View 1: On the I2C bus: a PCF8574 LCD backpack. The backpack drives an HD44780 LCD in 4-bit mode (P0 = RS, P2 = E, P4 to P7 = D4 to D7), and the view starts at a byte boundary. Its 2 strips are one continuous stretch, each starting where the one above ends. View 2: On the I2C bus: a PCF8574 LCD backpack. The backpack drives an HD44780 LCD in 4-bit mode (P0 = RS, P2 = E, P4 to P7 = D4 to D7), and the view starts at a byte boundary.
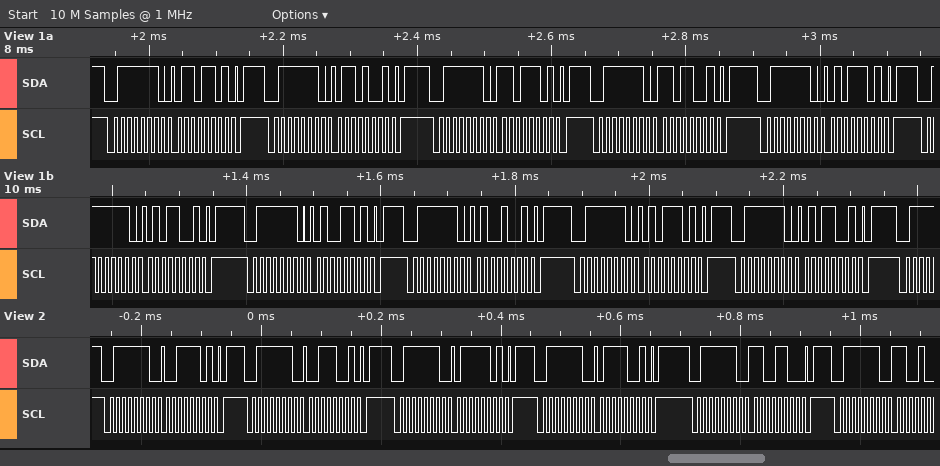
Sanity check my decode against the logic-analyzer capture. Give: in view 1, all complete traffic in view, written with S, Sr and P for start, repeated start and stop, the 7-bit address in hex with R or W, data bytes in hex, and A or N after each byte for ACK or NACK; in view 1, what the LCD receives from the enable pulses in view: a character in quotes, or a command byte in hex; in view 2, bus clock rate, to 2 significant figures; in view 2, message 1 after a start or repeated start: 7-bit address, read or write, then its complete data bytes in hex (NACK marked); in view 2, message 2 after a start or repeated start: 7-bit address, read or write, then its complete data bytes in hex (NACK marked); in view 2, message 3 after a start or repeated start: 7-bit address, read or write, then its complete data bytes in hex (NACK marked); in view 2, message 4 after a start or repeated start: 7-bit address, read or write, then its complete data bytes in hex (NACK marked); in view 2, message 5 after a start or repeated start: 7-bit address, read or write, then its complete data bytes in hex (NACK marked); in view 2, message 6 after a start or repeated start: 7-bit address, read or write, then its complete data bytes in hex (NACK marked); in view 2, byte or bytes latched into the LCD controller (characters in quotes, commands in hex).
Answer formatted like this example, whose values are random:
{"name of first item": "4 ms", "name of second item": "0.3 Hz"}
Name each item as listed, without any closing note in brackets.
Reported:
{"in view 1, all complete traffic in view, written with S, Sr and P for start, repeated start and stop, the 7-bit address in hex with R or W, data bytes in hex, and A or N after each byte for ACK or NACK": "S 3FW A 6D A P S 3FW A 69 A P S 3FW A DD A P S 3FW A D9 A P S 3FW A 5D A P S 3FW A 59 A P S 3FW A 4D A P S 3FW A 49 A P S 3FW A 5D A P S 3FW A 59 A P", "in view 1, what the LCD receives from the enable pulses in view: a character in quotes, or a command byte in hex": "'m' 'T'", "in view 2, bus clock rate, to 2 significant figures": "100 kHz", "in view 2, message 1 after a start or repeated start: 7-bit address, read or write, then its complete data bytes in hex": "0x3F write: 3D", "in view 2, message 2 after a start or repeated start: 7-bit address, read or write, then its complete data bytes in hex": "0x3F write: 39", "in view 2, message 3 after a start or repeated start: 7-bit address, read or write, then its complete data bytes in hex": "0x3F write: 7D", "in view 2, message 4 after a start or repeated start: 7-bit address, read or write, then its complete data bytes in hex": "0x3F write: 79", "in view 2, message 5 after a start or repeated start: 7-bit address, read or write, then its complete data bytes in hex": "0x3F write: CC", "in view 2, message 6 after a start or repeated start: 7-bit address, read or write, then its complete data bytes in hex": "0x3F write", "in view 2, byte or bytes latched into the LCD controller": "'7'"}
